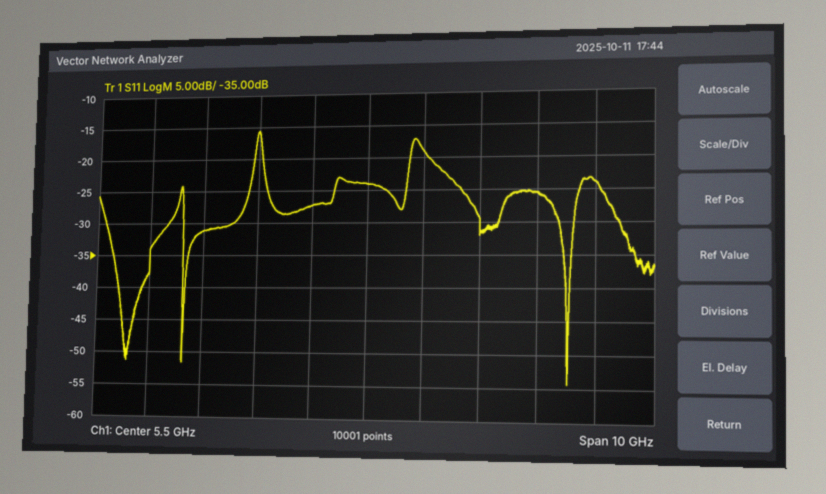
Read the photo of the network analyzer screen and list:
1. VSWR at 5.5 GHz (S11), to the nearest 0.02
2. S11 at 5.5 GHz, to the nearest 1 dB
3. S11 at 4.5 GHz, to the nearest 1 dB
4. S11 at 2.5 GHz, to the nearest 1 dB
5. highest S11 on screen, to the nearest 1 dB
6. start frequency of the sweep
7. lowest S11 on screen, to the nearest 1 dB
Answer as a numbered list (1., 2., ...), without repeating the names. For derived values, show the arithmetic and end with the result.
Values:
1. |Γ| = 10^(-24/20) = 0.0631; VSWR = (1 + 0.0631)/(1 − 0.0631) ≈ 1.13, so 1.14 to the nearest 0.02
2. -24 dB
3. -27 dB
4. -31 dB
5. -16 dB
6. 500 MHz
7. -54 dB
